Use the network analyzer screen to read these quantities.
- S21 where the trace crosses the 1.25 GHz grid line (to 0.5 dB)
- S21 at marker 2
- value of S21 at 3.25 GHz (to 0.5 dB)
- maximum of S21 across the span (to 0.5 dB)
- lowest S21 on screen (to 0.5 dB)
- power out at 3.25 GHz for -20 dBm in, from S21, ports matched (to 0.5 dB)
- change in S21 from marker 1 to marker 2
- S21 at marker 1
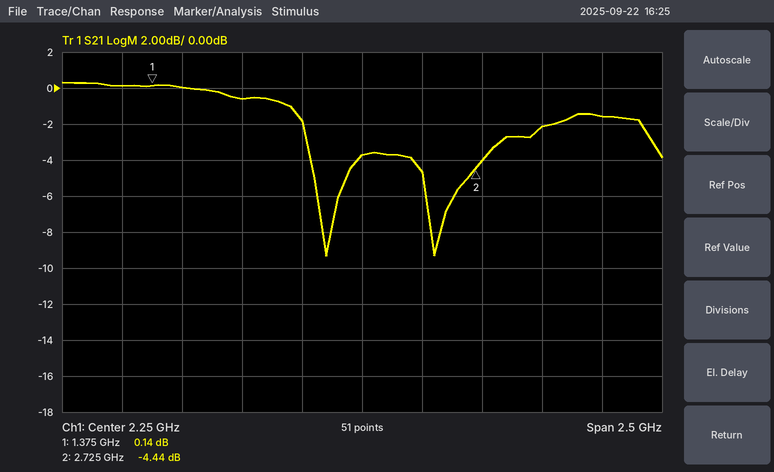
0.0 dB
-4.44 dB
-1.5 dB
0.5 dB
-9.5 dB
-21.5 dBm
-4.58 dB
0.14 dB
